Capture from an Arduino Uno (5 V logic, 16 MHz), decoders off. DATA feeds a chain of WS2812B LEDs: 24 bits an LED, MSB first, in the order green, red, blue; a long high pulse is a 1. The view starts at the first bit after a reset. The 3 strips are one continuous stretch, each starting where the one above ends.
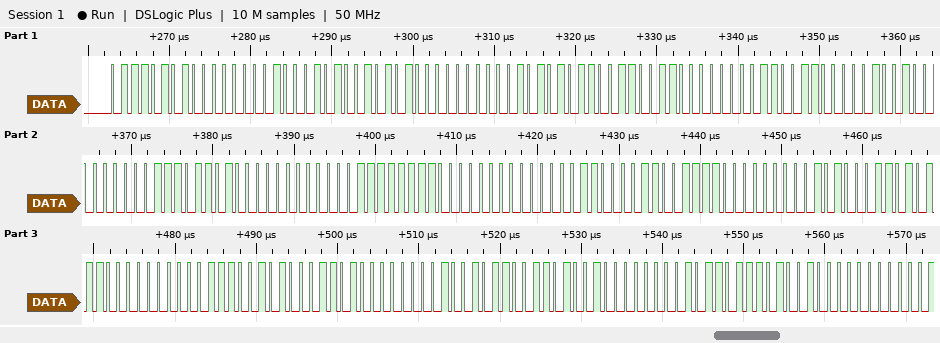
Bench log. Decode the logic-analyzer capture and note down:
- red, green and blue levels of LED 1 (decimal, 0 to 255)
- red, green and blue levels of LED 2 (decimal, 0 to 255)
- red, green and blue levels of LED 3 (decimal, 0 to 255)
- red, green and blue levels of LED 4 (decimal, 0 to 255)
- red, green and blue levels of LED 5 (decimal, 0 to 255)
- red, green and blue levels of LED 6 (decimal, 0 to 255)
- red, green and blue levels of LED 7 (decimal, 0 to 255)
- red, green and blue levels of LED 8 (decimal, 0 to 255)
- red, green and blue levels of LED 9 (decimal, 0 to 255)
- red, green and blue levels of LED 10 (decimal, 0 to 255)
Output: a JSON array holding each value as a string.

["0, 117, 138", "0, 84, 171", "0, 51, 204", "0, 18, 237", "15, 0, 240", "48, 0, 207", "81, 0, 174", "114, 0, 141", "150, 0, 105", "183, 0, 72"]
